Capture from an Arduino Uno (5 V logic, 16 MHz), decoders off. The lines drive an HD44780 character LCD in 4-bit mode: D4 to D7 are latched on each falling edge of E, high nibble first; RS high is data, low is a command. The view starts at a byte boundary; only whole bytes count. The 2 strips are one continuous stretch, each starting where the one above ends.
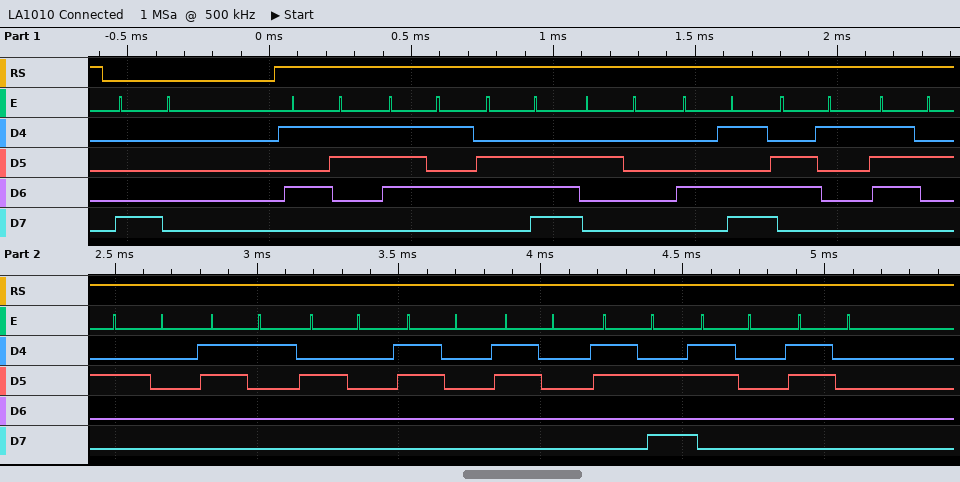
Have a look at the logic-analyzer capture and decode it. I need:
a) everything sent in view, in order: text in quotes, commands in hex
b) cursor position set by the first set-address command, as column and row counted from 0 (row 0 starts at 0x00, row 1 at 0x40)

0x80 "Sun Mar 1 00:00"
column 0, row 0
